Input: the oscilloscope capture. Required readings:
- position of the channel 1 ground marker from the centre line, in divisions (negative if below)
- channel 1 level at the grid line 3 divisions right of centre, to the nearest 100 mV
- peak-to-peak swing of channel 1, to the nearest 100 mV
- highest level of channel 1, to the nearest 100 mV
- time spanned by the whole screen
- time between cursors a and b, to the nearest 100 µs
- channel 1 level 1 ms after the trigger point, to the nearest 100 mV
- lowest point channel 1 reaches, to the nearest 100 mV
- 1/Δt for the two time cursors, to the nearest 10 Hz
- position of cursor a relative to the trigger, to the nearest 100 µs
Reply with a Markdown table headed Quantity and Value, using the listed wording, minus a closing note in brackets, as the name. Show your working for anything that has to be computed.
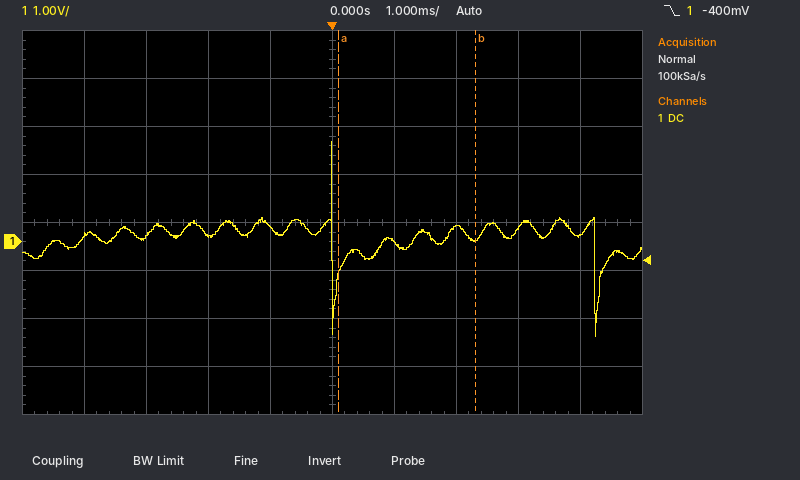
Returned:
| Quantity | Value |
|---|---|
| position of the channel 1 ground marker from the centre line, in divisions | -0.4 div |
| channel 1 level at the grid line 3 divisions right of centre, to the nearest 100 mV | 300 mV |
| peak-to-peak swing of channel 1, to the nearest 100 mV | 2.1 V − (-2.0 V) = 4.1 V |
| highest level of channel 1, to the nearest 100 mV | 2.1 V |
| time spanned by the whole screen | 10 ms |
| time between cursors a and b, to the nearest 100 µs | 2.2 ms |
| channel 1 level 1 ms after the trigger point, to the nearest 100 mV | 0.0 V |
| lowest point channel 1 reaches, to the nearest 100 mV | -2.0 V |
| 1/Δt for the two time cursors, to the nearest 10 Hz | 1 / 2.2 ms ≈ 450 Hz |
| position of cursor a relative to the trigger, to the nearest 100 µs | +100 µs |
